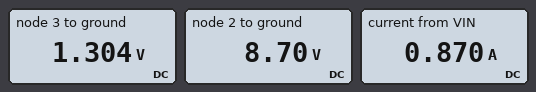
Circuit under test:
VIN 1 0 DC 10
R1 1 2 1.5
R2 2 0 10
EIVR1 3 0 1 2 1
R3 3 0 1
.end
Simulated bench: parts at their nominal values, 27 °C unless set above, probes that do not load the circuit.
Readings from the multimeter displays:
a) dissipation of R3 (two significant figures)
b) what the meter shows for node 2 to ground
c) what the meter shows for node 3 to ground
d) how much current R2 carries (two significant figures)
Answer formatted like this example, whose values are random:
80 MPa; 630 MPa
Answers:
1.7 W; 8.70 V; 1.304 V; 870 mA
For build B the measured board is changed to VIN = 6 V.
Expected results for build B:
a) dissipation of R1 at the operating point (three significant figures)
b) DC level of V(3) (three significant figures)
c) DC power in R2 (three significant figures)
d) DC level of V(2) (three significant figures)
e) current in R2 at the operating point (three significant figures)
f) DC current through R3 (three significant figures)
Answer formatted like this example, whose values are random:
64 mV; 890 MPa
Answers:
408 mW; 783 mV; 2.72 W; 5.22 V; 522 mA; 783 mA
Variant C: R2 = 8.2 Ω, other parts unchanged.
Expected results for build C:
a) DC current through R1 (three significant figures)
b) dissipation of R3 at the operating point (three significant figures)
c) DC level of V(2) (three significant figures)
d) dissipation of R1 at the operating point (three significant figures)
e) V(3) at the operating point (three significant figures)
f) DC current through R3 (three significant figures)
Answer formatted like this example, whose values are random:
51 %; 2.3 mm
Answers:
1.03 A; 2.39 W; 8.45 V; 1.59 W; 1.55 V; 1.55 A
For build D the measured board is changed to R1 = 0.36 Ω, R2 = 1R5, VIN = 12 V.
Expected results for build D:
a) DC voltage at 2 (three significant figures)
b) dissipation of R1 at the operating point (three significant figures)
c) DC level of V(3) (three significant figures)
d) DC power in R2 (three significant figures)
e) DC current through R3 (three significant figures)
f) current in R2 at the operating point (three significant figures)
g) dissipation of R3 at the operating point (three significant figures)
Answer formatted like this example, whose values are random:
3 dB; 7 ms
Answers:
9.68 V; 15.0 W; 2.32 V; 62.4 W; 2.32 A; 6.45 A; 5.39 W
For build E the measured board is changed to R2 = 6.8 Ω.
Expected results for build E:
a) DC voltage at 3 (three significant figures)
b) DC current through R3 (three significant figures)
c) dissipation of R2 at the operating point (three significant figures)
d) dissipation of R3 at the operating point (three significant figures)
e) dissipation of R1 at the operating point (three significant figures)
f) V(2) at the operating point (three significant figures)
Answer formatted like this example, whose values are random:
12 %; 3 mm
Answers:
1.81 V; 1.81 A; 9.87 W; 3.27 W; 2.18 W; 8.19 V
